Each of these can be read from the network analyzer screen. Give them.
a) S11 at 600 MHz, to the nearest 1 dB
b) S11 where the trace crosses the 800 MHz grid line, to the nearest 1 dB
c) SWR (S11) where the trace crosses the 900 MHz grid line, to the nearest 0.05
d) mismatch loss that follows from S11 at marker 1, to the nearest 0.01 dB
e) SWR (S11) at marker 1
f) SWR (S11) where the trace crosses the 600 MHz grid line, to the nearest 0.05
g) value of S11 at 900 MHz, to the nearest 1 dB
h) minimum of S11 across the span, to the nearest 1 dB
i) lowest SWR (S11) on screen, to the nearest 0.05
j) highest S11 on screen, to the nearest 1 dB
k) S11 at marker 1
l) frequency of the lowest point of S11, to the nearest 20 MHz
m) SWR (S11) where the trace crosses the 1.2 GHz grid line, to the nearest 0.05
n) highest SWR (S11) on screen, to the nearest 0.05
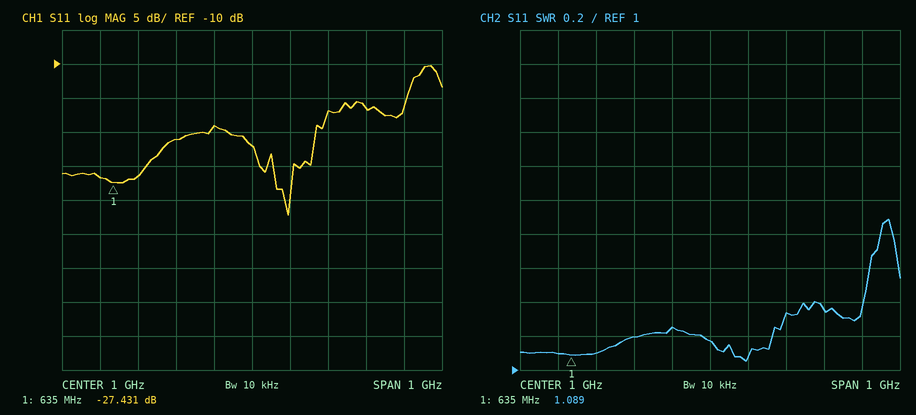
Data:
-27 dB
-21 dB
1.25
0.01 dB
1.089
1.10
-19 dB
-32 dB
1.05
-10 dB
-27.431 dB
1.10 GHz
1.35
1.90
